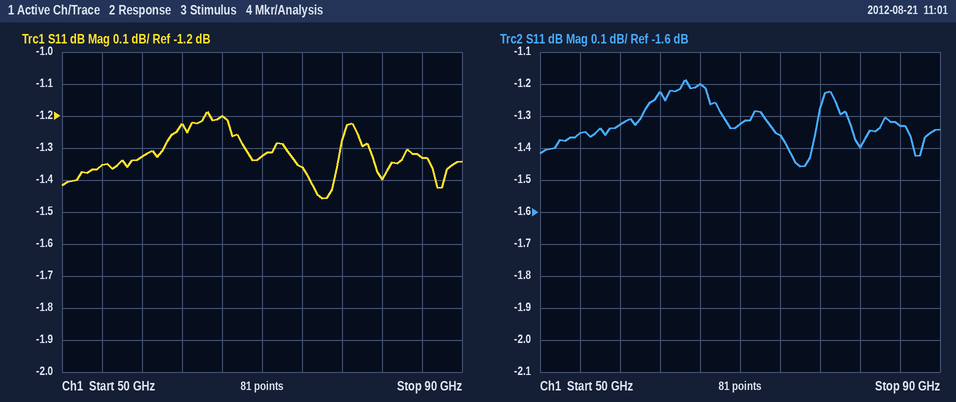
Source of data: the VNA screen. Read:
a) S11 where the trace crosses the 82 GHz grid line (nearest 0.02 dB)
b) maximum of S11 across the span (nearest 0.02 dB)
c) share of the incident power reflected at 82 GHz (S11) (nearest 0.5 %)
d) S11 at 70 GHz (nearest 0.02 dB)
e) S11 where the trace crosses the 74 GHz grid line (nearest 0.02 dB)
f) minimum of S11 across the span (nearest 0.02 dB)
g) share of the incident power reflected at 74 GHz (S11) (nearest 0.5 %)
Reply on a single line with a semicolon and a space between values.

-1.40 dB; -1.18 dB; 72.5 %; -1.32 dB; -1.36 dB; -1.46 dB; 73.0 %
